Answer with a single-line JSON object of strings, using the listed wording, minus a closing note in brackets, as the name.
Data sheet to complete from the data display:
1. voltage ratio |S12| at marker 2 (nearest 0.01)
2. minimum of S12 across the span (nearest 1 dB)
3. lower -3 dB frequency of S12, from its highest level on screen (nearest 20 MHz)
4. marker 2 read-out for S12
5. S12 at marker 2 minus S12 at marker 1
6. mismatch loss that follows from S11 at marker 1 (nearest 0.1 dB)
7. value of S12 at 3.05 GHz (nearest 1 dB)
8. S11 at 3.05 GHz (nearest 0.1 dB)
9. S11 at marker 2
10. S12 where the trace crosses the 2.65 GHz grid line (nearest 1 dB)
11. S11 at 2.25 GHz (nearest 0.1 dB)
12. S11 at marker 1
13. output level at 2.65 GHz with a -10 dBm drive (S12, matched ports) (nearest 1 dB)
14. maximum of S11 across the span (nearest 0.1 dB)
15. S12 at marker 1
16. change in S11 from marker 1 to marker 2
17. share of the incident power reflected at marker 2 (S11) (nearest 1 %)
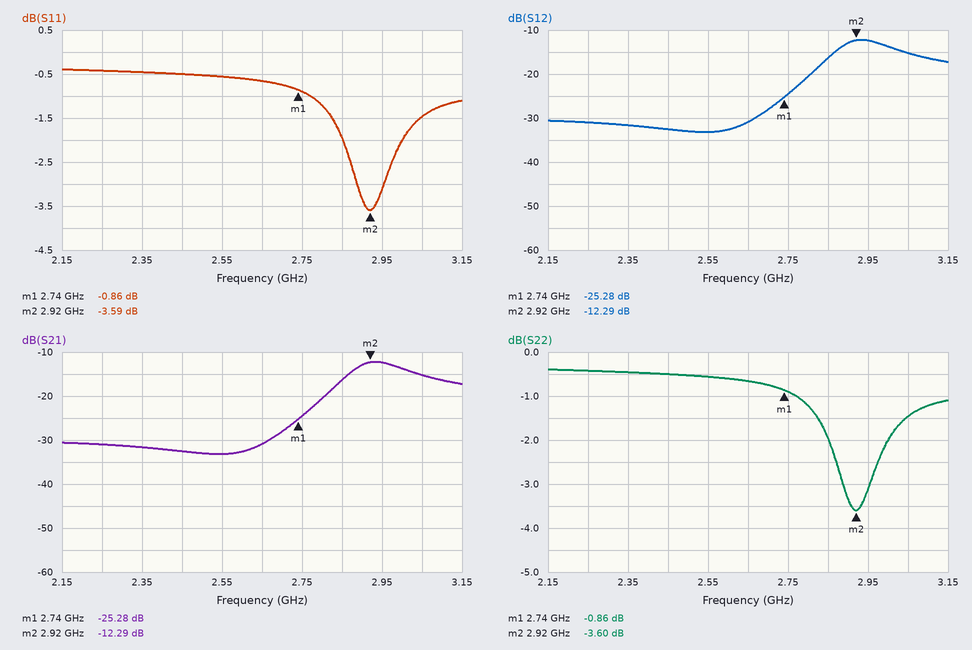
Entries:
{"voltage ratio |S12| at marker 2": "0.24", "minimum of S12 across the span": "-33 dB", "lower -3 dB frequency of S12, from its highest level on screen": "2.86 GHz", "marker 2 read-out for S12": "-12.29 dB", "S12 at marker 2 minus S12 at marker 1": "12.99 dB", "mismatch loss that follows from S11 at marker 1": "7.5 dB", "value of S12 at 3.05 GHz": "-15 dB", "S11 at 3.05 GHz": "-1.5 dB", "S11 at marker 2": "-3.59 dB", "S12 where the trace crosses the 2.65 GHz grid line": "-31 dB", "S11 at 2.25 GHz": "-0.4 dB", "S11 at marker 1": "-0.86 dB", "output level at 2.65 GHz with a -10 dBm drive (S12, matched ports)": "-41 dBm", "maximum of S11 across the span": "-0.4 dB", "S12 at marker 1": "-25.28 dB", "change in S11 from marker 1 to marker 2": "-2.73 dB", "share of the incident power reflected at marker 2 (S11)": "44 %"}
